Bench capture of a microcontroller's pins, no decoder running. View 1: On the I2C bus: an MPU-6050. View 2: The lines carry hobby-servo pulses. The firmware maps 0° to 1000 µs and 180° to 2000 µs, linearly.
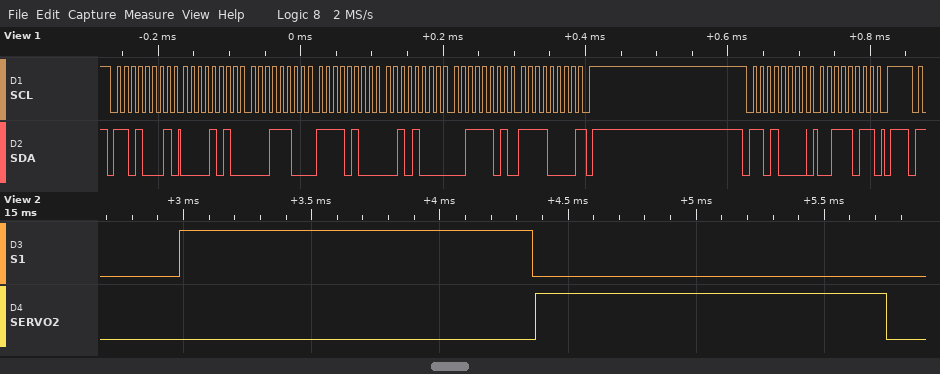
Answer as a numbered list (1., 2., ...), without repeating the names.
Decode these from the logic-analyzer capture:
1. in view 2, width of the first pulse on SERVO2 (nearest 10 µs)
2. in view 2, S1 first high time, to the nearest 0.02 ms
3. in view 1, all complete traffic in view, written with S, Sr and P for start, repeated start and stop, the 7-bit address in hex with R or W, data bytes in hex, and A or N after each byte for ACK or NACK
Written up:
1. 1370 µs
2. 1.38 ms
3. S 68R A 0A A 1C A F4 A 28 A 3D A F0 N P S 68W A 3B A P
